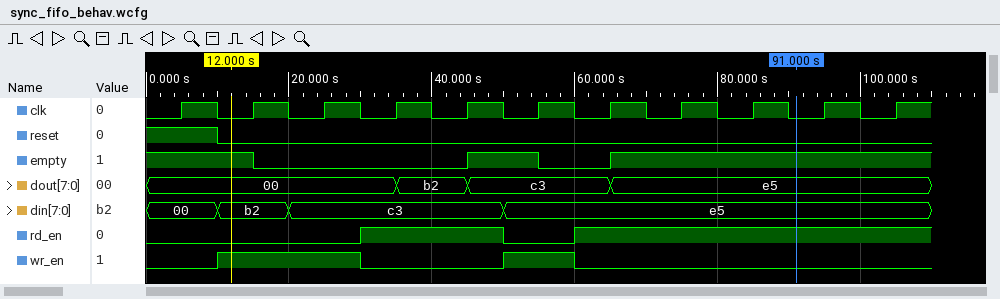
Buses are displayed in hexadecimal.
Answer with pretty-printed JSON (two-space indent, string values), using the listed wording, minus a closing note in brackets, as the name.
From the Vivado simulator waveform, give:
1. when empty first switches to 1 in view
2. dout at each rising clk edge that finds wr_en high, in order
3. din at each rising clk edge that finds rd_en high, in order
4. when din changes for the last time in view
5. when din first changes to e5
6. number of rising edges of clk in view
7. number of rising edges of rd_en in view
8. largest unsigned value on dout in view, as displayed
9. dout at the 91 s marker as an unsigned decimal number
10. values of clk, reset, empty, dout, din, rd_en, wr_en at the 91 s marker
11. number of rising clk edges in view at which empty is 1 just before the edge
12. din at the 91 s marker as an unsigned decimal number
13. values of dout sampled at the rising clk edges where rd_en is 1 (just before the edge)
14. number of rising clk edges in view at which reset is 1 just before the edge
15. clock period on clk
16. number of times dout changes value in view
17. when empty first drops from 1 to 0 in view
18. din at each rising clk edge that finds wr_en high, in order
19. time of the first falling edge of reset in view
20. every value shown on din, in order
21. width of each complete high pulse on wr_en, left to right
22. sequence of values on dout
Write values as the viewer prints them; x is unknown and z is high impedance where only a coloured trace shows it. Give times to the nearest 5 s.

{
  "when empty first switches to 1 in view": "45 s",
  "dout at each rising clk edge that finds wr_en high, in order": "00, 00, c3",
  "din at each rising clk edge that finds rd_en high, in order": "c3, c3, e5, e5, e5, e5, e5",
  "when din changes for the last time in view": "50 s",
  "when din first changes to e5": "50 s",
  "number of rising edges of clk in view": "11",
  "number of rising edges of rd_en in view": "2",
  "largest unsigned value on dout in view, as displayed": "e5",
  "dout at the 91 s marker as an unsigned decimal number": "229",
  "values of clk, reset, empty, dout, din, rd_en, wr_en at the 91 s marker": "clk=0, reset=0, empty=1, dout=e5, din=e5, rd_en=1, wr_en=0",
  "number of rising clk edges in view at which empty is 1 just before the edge": "7",
  "din at the 91 s marker as an unsigned decimal number": "229",
  "values of dout sampled at the rising clk edges where rd_en is 1": "00, b2, c3, e5, e5, e5, e5",
  "number of rising clk edges in view at which reset is 1 just before the edge": "1",
  "clock period on clk": "10 s",
  "number of times dout changes value in view": "3",
  "when empty first drops from 1 to 0 in view": "15 s",
  "din at each rising clk edge that finds wr_en high, in order": "b2, c3, e5",
  "time of the first falling edge of reset in view": "10 s",
  "every value shown on din, in order": "00, b2, c3, e5",
  "width of each complete high pulse on wr_en, left to right": "20 s, 10 s",
  "sequence of values on dout": "00, b2, c3, e5"
}
